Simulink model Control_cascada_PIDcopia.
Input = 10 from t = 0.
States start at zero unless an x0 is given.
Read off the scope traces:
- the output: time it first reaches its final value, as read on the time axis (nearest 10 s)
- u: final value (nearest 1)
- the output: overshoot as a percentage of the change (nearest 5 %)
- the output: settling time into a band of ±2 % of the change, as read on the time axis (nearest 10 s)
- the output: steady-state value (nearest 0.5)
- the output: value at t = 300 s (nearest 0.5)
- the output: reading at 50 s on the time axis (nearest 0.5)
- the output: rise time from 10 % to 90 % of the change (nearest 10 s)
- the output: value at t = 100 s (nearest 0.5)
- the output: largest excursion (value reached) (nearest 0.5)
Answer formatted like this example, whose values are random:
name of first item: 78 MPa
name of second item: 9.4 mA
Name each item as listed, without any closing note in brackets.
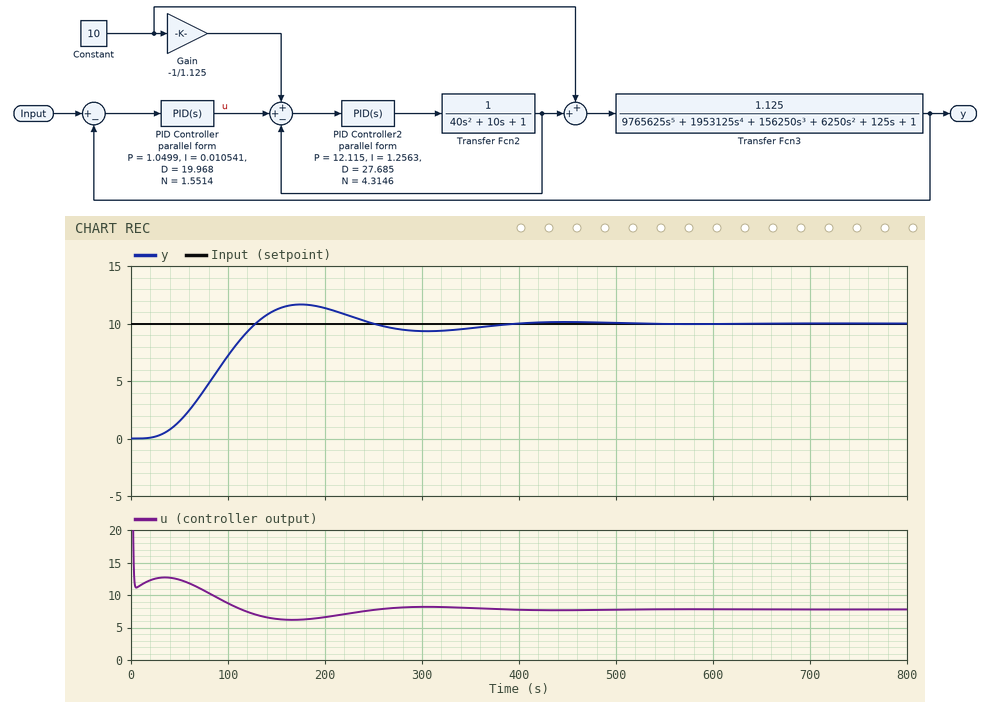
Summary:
the output: time it first reaches its final value, as read on the time axis: 130 s
u: final value: 8
the output: overshoot as a percentage of the change: 15 %
the output: settling time into a band of ±2 % of the change, as read on the time axis: 370 s
the output: steady-state value: 10.0
the output: value at t = 300 s: 9.5
the output: reading at 50 s on the time axis: 1.5
the output: rise time from 10 % to 90 % of the change: 70 s
the output: value at t = 100 s: 7.0
the output: largest excursion (value reached): 11.5
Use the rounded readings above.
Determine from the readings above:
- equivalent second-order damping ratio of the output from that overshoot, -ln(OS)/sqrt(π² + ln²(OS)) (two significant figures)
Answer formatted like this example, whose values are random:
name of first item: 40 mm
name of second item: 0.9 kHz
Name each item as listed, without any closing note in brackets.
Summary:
equivalent second-order damping ratio of the output from that overshoot, -ln(OS)/sqrt(π² + ln²(OS)): 0.52
